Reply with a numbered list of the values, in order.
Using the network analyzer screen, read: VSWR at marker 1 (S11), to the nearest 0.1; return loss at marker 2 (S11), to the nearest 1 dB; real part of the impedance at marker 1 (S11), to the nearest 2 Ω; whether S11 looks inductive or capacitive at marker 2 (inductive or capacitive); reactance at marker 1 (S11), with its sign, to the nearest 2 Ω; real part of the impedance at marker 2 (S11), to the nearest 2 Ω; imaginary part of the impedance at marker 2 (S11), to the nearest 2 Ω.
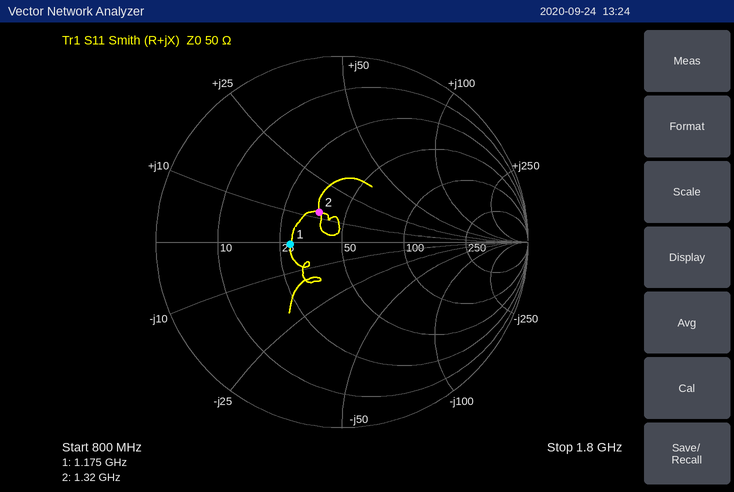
1. 1.8
2. 14 dB
3. 28 Ω
4. inductive
5. 0 Ω
6. 38 Ω
7. +12 Ω
